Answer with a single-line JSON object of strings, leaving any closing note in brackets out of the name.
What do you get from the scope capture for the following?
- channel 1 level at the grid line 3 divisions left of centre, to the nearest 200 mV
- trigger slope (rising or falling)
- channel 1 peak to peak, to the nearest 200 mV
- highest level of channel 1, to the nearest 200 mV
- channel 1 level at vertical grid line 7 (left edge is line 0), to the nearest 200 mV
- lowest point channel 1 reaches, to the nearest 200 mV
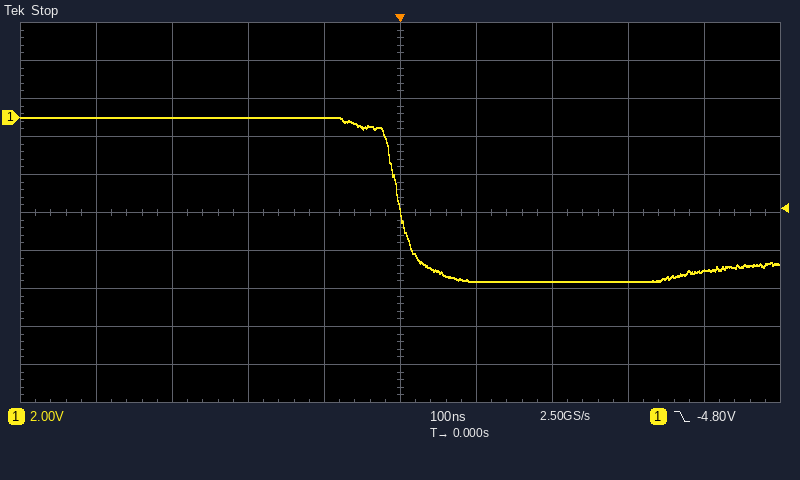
{"channel 1 level at the grid line 3 divisions left of centre, to the nearest 200 mV": "0.0 V", "trigger slope": "falling", "channel 1 peak to peak, to the nearest 200 mV": "8.6 V", "highest level of channel 1, to the nearest 200 mV": "0.0 V", "channel 1 level at vertical grid line 7 (left edge is line 0), to the nearest 200 mV": "-8.6 V", "lowest point channel 1 reaches, to the nearest 200 mV": "-8.6 V"}
